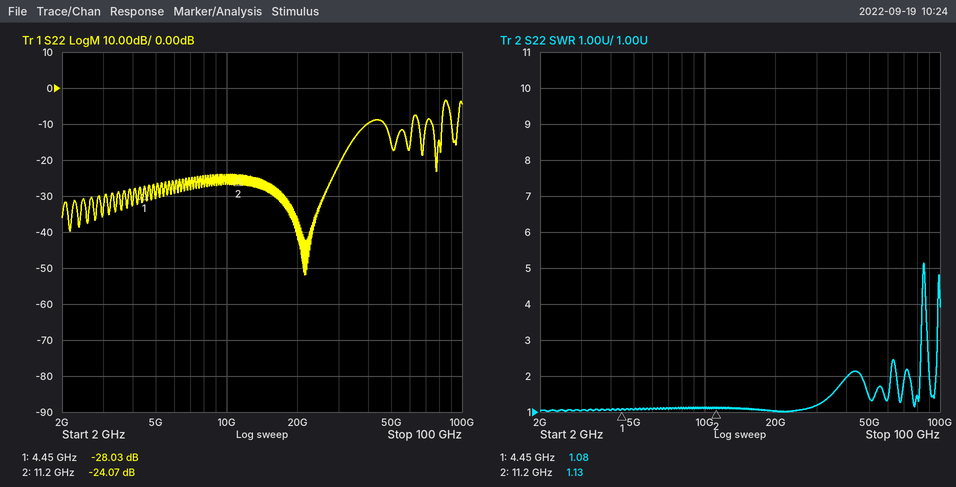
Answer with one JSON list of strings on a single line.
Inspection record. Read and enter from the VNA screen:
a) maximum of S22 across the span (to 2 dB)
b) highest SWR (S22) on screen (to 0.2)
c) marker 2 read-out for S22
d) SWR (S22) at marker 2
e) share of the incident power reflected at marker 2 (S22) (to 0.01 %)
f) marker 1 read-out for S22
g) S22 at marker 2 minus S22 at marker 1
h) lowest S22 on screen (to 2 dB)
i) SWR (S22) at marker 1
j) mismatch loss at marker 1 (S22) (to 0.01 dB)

["-4 dB", "5.2", "-24.07 dB", "1.13", "0.39 %", "-28.03 dB", "3.96 dB", "-52 dB", "1.08", "0.01 dB"]
